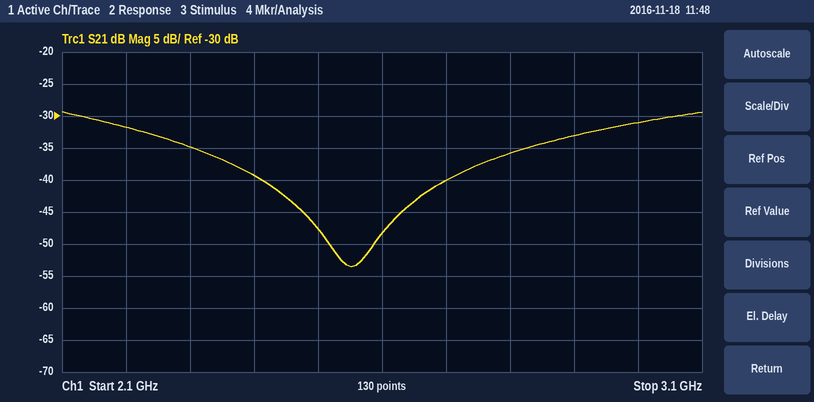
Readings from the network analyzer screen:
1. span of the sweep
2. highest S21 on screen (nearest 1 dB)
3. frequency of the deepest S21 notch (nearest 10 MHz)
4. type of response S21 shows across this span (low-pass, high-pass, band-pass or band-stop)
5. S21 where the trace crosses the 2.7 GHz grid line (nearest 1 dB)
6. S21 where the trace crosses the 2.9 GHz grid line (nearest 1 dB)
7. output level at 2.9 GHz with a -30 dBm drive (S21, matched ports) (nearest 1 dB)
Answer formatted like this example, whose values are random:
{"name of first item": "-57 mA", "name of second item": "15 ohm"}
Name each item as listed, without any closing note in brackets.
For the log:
{"span of the sweep": "1 GHz", "highest S21 on screen": "-29 dB", "frequency of the deepest S21 notch": "2.55 GHz", "type of response S21 shows across this span": "band-stop", "S21 where the trace crosses the 2.7 GHz grid line": "-40 dB", "S21 where the trace crosses the 2.9 GHz grid line": "-33 dB", "output level at 2.9 GHz with a -30 dBm drive (S21, matched ports)": "-63 dBm"}
